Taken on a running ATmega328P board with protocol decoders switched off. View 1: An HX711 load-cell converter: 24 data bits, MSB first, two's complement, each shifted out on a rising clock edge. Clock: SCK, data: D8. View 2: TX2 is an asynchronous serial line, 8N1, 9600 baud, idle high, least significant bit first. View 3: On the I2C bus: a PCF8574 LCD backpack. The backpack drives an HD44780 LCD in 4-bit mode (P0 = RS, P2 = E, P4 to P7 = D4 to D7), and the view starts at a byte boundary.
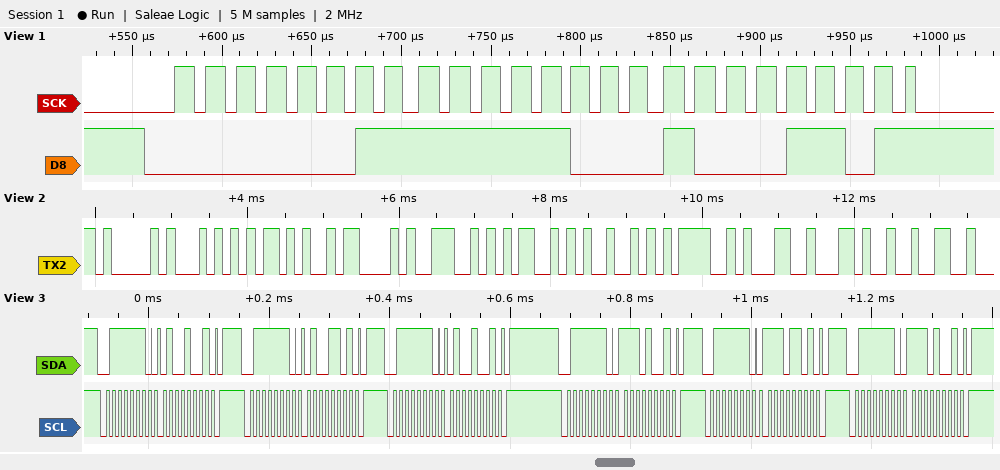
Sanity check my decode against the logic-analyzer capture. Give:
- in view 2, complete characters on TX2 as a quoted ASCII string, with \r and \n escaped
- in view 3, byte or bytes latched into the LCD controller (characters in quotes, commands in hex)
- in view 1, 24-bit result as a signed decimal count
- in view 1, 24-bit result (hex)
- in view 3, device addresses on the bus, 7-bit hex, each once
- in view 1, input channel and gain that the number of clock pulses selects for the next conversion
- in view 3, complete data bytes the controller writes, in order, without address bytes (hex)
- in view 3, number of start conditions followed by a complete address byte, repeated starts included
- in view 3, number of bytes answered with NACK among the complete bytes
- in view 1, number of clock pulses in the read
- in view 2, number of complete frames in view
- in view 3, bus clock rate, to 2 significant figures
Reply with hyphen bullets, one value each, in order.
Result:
- "AT+CNMI=1,2"
- 'N'
- 260237
- 0x03F88D
- 0x3F
- channel A, gain 128
- 49 4D 49 E9 ED E9
- 6
- 0
- 25
- 11
- 100 kHz
